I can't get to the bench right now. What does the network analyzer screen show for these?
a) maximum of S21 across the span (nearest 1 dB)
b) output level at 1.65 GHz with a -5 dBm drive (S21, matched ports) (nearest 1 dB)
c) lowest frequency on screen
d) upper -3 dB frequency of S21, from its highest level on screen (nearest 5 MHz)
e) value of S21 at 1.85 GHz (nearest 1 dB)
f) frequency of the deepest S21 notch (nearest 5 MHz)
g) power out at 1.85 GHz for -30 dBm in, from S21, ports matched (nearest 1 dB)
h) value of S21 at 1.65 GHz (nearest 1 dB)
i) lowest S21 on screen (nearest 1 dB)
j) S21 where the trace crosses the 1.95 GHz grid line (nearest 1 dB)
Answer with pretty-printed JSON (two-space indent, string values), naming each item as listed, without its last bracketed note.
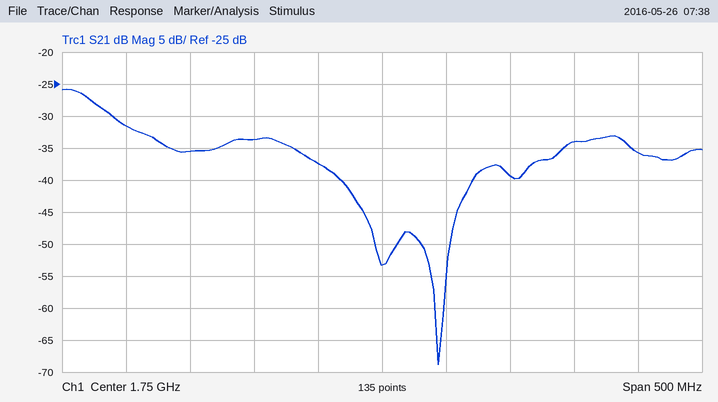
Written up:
{
  "maximum of S21 across the span": "-26 dB",
  "output level at 1.65 GHz with a -5 dBm drive (S21, matched ports)": "-39 dBm",
  "lowest frequency on screen": "1.5 GHz",
  "upper -3 dB frequency of S21, from its highest level on screen": "1.530 GHz",
  "value of S21 at 1.85 GHz": "-39 dB",
  "frequency of the deepest S21 notch": "1.795 GHz",
  "power out at 1.85 GHz for -30 dBm in, from S21, ports matched": "-69 dBm",
  "value of S21 at 1.65 GHz": "-34 dB",
  "lowest S21 on screen": "-69 dB",
  "S21 where the trace crosses the 1.95 GHz grid line": "-36 dB"
}
